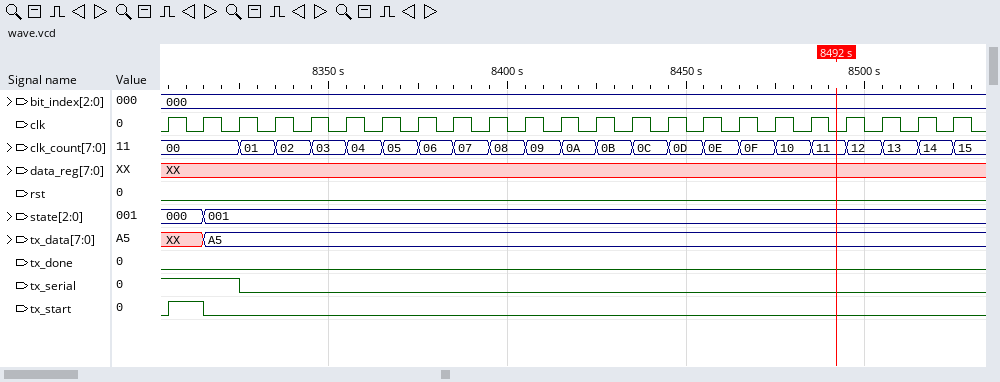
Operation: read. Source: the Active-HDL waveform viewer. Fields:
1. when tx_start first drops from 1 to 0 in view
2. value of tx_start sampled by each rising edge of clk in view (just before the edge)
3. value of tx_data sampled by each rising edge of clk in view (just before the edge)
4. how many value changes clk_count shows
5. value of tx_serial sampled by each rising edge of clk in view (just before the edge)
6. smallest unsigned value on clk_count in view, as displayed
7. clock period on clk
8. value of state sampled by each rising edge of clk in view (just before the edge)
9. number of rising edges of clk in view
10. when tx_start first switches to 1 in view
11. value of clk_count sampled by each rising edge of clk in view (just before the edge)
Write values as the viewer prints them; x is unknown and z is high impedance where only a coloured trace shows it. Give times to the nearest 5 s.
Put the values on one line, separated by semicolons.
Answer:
8315 s; 0 1 0 0 0 0 0 0 0 0 0 0 0 0 0 0 0 0 0 0 0 0 0; XX, XX, A5, A5, A5, A5, A5, A5, A5, A5, A5, A5, A5, A5, A5, A5, A5, A5, A5, A5, A5, A5, A5; 21; 1 1 1 0 0 0 0 0 0 0 0 0 0 0 0 0 0 0 0 0 0 0 0; 00; 10 s; 000, 000, 001, 001, 001, 001, 001, 001, 001, 001, 001, 001, 001, 001, 001, 001, 001, 001, 001, 001, 001, 001, 001; 23; 8305 s; 00, 00, 00, 01, 02, 03, 04, 05, 06, 07, 08, 09, 0A, 0B, 0C, 0D, 0E, 0F, 10, 11, 12, 13, 14
